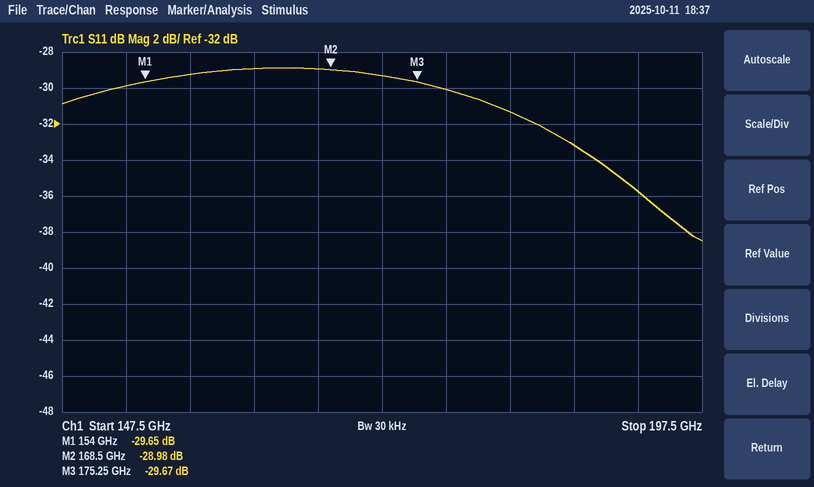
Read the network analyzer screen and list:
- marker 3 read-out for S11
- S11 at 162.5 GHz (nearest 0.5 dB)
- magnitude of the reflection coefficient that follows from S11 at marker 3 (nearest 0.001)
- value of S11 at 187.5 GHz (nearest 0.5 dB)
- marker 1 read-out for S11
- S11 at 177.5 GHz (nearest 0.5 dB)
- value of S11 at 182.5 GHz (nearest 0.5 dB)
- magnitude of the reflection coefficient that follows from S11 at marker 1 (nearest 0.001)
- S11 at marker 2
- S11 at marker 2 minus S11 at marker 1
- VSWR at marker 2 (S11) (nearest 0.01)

-29.67 dB
-29.0 dB
0.033
-33.0 dB
-29.65 dB
-30.0 dB
-31.5 dB
0.033
-28.98 dB
0.67 dB
1.07
